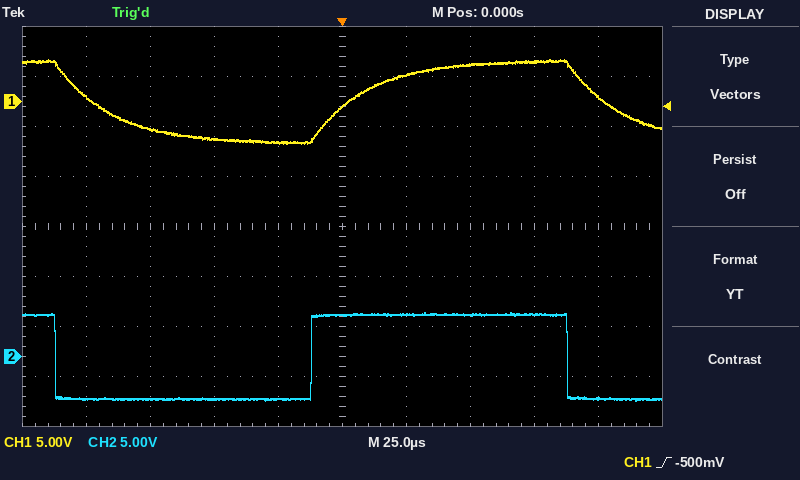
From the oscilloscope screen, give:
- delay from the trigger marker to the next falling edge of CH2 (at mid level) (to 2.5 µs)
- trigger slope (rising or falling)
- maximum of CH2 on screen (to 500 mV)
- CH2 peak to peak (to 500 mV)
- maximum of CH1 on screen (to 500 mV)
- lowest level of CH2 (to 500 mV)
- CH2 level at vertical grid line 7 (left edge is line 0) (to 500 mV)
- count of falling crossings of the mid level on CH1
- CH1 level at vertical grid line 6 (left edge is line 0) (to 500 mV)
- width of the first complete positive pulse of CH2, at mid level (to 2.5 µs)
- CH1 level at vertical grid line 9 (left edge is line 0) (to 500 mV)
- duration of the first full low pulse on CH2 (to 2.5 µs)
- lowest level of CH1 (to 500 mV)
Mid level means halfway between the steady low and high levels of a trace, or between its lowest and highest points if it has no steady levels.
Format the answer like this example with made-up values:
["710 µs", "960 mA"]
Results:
["87.5 µs", "rising", "4.5 V", "9.0 V", "4.0 V", "-4.5 V", "4.0 V", "2", "2.5 V", "100.0 µs", "500 mV", "100.0 µs", "-4.0 V"]
